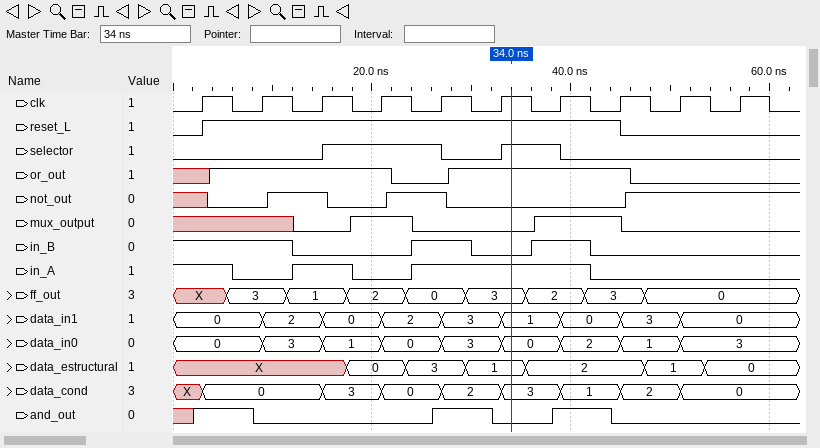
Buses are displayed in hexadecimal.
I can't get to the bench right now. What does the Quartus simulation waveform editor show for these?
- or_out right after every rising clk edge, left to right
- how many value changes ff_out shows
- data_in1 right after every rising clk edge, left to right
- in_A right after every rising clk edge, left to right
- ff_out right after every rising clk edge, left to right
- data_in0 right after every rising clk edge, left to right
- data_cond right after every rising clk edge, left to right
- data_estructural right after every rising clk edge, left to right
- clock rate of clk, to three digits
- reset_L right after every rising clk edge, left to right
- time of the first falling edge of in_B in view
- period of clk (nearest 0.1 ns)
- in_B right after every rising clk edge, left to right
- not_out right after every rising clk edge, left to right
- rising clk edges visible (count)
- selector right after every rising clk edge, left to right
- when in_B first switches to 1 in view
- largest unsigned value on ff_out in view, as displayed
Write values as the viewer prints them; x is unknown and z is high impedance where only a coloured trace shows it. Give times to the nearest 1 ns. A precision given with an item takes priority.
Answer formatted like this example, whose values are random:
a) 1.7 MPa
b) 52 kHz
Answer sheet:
a) x 1 1 1 0 1 1 1 0 0
b) 8
c) 0, 2, 0, 2, 3, 1, 0, 3, 0, 0
d) 1 0 1 0 1 1 1 0 0 0
e) X, 3, 1, 2, 0, 3, 2, 3, 0, 0
f) 0, 3, 1, 0, 3, 0, 2, 1, 3, 3
g) 0, 0, 3, 0, 2, 3, 1, 2, 0, 0
h) X, X, X, 0, 3, 1, 2, 2, 1, 0
i) 167 MHz
j) 1 1 1 1 1 1 1 0 0 0
k) 12 ns
l) 6 ns
m) 1 1 0 0 1 0 1 0 0 0
n) x 0 1 0 1 0 0 0 1 1
o) 10
p) 0 0 1 1 0 1 0 0 0 0
q) 24 ns
r) 3
